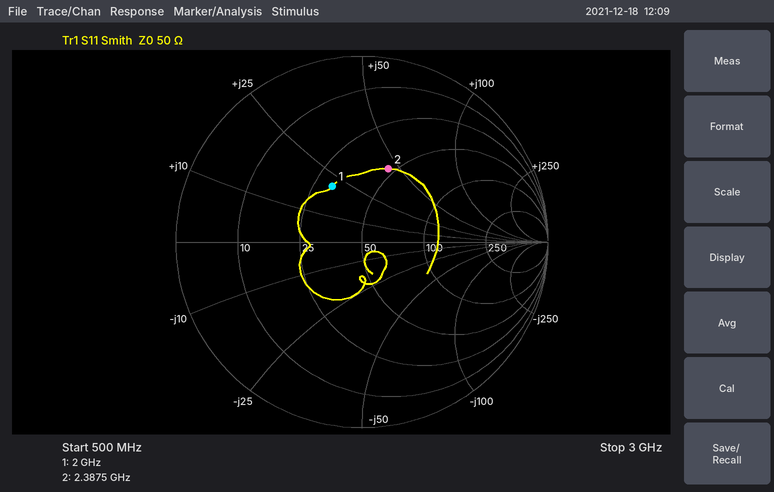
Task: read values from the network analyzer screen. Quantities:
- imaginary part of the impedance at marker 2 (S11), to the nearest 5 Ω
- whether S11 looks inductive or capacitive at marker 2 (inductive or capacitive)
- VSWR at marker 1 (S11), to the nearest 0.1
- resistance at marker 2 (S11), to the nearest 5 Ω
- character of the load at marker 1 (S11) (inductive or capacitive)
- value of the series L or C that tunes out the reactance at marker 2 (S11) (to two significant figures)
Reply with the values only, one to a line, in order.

+45 Ω
inductive
2.0
45 Ω
inductive
1.5 pF
